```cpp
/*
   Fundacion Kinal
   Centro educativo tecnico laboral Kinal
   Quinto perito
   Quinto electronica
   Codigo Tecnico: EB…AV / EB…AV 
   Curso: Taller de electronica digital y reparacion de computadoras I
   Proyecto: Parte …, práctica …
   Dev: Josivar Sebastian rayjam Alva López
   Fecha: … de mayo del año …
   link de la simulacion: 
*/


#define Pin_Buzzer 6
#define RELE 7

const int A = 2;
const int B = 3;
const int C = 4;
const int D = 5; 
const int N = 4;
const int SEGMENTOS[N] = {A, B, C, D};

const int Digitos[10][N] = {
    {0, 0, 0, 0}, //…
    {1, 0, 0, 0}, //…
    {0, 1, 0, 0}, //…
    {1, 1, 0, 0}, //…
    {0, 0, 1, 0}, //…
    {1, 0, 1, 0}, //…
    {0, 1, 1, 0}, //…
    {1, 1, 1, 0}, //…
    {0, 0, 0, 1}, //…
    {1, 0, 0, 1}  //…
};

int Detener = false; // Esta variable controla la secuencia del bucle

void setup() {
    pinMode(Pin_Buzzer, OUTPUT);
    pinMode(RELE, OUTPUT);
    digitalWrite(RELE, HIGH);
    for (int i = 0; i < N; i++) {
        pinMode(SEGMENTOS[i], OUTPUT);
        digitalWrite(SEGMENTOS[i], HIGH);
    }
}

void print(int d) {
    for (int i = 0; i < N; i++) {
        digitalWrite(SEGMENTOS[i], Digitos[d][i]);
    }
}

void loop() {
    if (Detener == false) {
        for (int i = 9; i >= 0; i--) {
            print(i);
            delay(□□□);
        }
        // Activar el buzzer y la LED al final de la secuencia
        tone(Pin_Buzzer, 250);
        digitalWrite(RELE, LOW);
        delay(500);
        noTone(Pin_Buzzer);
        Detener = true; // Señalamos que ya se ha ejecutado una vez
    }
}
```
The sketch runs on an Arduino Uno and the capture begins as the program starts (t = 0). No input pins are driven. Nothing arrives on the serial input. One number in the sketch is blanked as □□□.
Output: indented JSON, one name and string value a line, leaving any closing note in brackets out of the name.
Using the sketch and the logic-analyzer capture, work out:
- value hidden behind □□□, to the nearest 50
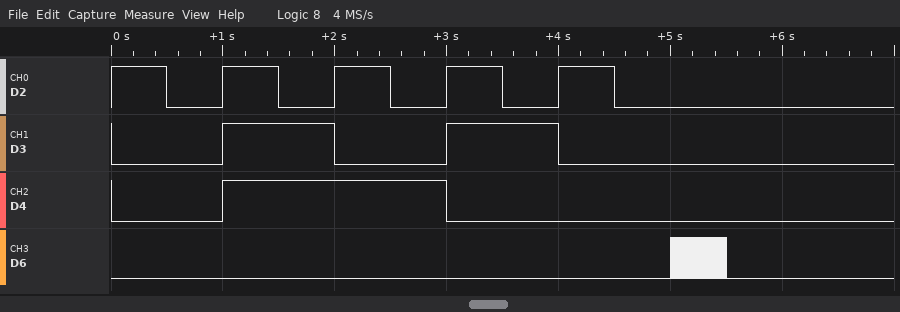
{
  "value hidden behind □□□, to the nearest 50": "500"
}
